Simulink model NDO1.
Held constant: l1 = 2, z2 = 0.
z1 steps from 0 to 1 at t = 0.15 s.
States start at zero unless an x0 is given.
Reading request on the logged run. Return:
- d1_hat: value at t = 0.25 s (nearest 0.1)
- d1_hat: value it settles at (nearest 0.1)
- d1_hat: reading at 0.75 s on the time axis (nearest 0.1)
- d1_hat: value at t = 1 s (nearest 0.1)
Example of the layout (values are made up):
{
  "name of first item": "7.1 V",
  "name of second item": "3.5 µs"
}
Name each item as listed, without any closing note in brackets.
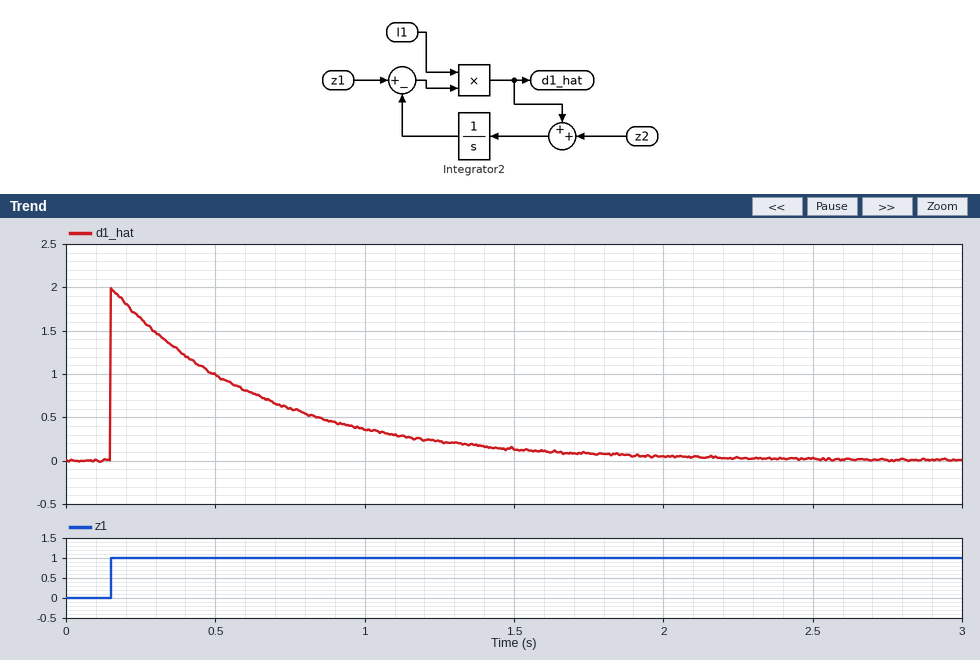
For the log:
{
  "d1_hat: value at t = 0.25 s": "1.6",
  "d1_hat: value it settles at": "0.0",
  "d1_hat: reading at 0.75 s on the time axis": "0.6",
  "d1_hat: value at t = 1 s": "0.4"
}
